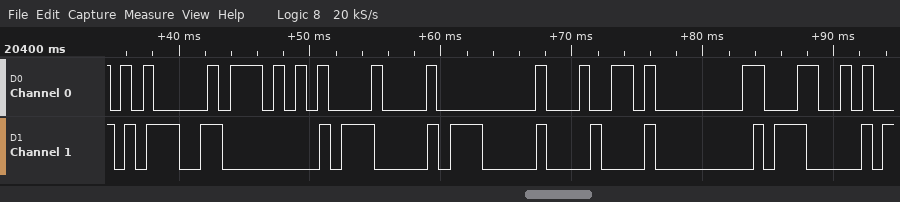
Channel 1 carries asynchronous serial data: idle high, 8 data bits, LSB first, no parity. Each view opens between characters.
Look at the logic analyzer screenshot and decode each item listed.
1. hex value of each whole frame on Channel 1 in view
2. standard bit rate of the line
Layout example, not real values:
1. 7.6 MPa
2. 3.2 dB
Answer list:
1. 9D, 00, 07, 07, 08, 00, 07
2. 1200 baud
